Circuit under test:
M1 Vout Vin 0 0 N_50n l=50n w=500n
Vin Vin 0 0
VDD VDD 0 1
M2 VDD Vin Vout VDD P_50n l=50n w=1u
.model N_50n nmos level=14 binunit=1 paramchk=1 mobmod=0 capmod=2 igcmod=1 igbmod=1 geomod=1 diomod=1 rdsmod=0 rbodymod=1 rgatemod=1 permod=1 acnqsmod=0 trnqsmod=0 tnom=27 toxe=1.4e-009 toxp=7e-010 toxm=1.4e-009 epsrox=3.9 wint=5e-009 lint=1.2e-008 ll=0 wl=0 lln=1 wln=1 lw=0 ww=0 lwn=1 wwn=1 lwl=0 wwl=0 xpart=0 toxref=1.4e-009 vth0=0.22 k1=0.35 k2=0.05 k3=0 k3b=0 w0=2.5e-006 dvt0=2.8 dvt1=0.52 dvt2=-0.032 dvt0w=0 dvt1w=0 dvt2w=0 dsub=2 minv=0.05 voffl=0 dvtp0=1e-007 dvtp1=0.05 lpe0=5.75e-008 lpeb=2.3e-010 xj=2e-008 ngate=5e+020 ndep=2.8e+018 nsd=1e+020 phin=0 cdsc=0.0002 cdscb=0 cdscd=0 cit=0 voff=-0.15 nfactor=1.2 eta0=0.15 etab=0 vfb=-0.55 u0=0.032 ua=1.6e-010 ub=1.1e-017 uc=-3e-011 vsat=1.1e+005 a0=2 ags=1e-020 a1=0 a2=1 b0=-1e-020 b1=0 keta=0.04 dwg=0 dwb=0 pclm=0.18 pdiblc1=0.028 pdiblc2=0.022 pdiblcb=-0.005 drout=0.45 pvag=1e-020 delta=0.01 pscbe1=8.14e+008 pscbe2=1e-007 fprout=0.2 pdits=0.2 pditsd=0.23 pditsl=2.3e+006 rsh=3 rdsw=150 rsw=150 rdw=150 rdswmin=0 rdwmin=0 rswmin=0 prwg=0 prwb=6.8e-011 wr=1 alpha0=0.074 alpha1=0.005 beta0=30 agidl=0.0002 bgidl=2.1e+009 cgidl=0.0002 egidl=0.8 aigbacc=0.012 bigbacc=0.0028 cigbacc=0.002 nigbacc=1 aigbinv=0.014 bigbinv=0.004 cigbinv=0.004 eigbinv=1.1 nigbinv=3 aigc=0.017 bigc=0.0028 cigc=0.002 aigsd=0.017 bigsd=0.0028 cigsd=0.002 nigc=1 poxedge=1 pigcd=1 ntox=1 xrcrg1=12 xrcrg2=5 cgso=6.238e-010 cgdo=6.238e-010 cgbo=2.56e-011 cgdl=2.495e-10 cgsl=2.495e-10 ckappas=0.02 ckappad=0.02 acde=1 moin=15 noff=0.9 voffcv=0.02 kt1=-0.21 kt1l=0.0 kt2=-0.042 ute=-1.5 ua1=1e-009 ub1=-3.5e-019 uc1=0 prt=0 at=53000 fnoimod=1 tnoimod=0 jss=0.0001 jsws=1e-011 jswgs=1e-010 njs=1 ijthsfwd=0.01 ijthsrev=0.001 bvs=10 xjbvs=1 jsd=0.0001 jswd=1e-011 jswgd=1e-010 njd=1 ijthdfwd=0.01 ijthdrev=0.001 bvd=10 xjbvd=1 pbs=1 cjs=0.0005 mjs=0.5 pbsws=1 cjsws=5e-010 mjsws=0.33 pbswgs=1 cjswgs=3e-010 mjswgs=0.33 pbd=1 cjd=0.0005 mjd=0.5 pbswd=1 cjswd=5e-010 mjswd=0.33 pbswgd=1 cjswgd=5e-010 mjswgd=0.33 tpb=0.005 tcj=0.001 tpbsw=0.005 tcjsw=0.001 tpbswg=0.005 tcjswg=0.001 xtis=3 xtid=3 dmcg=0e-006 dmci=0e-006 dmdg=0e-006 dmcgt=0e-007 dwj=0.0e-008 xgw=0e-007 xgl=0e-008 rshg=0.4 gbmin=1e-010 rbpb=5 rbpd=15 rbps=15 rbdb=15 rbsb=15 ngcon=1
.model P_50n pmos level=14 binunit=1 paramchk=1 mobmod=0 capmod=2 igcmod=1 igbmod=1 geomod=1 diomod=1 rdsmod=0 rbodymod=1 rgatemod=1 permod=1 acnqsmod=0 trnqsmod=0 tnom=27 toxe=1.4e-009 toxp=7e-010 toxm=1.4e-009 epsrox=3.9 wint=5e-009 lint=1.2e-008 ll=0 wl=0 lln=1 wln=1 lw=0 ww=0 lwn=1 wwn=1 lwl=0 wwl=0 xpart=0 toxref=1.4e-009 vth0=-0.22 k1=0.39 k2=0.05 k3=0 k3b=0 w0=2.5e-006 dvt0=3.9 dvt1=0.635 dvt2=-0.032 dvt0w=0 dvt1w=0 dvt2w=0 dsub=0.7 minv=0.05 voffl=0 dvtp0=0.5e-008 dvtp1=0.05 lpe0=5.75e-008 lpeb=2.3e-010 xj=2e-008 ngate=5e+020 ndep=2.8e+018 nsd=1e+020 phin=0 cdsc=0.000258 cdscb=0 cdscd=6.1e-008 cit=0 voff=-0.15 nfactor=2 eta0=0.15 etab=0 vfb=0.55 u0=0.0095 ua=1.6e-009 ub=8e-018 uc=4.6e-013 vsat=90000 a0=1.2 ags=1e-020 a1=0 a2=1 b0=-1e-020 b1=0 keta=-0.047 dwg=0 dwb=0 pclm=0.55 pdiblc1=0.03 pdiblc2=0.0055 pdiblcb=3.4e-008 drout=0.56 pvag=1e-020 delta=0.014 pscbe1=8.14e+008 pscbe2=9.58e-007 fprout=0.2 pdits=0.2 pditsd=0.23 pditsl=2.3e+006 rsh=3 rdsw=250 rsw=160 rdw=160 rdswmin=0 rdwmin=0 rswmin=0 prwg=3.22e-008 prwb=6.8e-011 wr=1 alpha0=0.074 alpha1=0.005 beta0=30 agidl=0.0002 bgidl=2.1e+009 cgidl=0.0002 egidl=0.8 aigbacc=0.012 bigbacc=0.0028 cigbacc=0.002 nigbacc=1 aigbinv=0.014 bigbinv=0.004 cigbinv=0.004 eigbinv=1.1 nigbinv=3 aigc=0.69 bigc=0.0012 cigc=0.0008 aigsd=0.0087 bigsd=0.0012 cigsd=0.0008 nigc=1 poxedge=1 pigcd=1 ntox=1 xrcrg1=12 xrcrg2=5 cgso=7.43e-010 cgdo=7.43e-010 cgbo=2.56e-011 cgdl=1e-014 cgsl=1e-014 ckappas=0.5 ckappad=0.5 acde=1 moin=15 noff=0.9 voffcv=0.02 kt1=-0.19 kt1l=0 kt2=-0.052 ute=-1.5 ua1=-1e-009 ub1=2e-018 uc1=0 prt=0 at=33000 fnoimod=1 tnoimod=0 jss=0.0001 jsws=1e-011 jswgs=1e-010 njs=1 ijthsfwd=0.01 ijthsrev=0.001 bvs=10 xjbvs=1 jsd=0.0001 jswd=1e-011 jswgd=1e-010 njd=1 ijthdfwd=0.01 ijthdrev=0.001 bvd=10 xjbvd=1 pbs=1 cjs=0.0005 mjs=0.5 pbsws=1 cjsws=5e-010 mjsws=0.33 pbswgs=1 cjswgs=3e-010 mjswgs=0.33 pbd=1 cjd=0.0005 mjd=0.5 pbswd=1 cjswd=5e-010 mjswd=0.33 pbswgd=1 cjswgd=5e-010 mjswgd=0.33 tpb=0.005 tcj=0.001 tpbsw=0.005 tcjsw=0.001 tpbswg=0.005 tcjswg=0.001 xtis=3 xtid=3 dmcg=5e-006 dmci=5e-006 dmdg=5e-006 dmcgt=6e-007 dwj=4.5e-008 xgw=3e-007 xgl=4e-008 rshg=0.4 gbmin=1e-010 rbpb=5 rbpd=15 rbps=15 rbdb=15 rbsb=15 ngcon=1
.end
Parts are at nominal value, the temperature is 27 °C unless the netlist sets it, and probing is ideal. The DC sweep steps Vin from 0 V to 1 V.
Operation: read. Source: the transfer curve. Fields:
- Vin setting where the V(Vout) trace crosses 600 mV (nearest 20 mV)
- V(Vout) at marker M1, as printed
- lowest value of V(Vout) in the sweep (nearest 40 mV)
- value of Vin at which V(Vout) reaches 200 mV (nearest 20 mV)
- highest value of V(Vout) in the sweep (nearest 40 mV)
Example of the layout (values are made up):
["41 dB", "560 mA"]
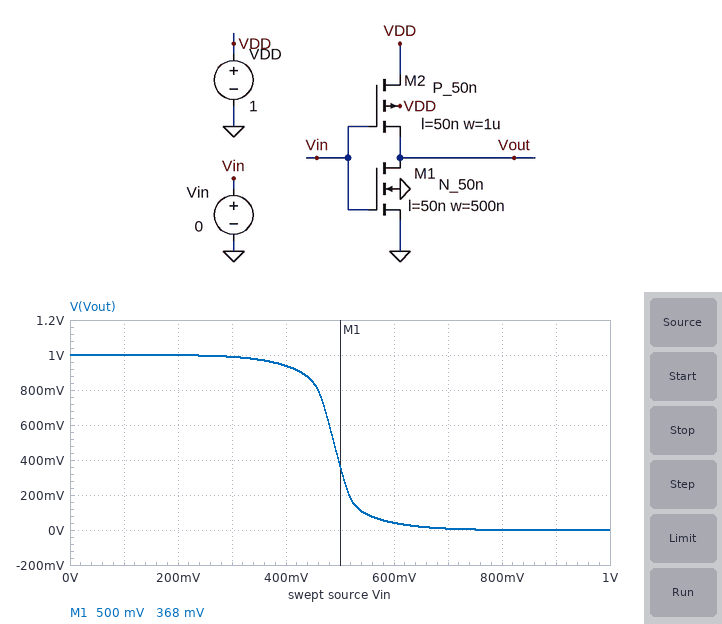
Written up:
["480 mV", "368 mV", "0 V", "520 mV", "1.00 V"]
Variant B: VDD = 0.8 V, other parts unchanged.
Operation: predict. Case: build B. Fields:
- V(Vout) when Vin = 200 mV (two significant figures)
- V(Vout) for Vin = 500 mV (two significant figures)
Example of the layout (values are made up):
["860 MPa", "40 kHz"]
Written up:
["800 mV", "10 mV"]
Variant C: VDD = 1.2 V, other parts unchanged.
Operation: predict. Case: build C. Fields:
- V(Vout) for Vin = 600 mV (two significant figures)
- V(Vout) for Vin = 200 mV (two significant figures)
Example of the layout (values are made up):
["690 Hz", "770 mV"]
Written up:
["470 mV", "1.2 V"]
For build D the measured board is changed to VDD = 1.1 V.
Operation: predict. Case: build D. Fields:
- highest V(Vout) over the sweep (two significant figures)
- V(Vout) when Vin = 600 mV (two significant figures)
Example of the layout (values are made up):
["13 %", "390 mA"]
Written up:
["1.1 V", "130 mV"]
